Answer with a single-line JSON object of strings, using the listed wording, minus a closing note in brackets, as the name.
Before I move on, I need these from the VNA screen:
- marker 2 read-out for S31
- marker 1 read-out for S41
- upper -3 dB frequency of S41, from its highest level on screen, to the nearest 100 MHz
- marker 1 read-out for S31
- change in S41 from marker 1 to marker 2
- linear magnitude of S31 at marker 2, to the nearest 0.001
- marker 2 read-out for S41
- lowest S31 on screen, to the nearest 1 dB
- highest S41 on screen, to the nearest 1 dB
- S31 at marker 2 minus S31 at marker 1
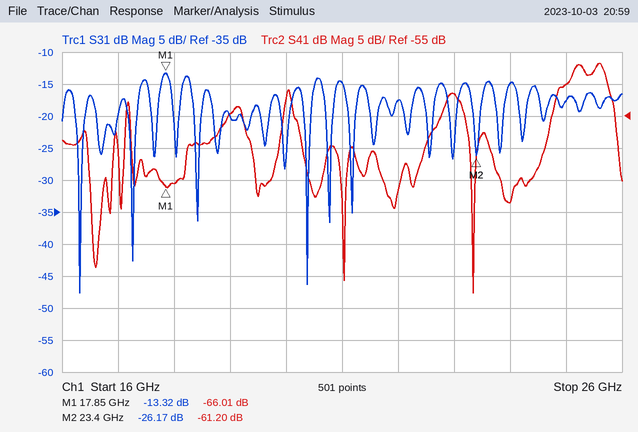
{"marker 2 read-out for S31": "-26.17 dB", "marker 1 read-out for S41": "-66.01 dB", "upper -3 dB frequency of S41, from its highest level on screen, to the nearest 100 MHz": "25.7 GHz", "marker 1 read-out for S31": "-13.32 dB", "change in S41 from marker 1 to marker 2": "4.81 dB", "linear magnitude of S31 at marker 2, to the nearest 0.001": "0.049", "marker 2 read-out for S41": "-61.20 dB", "lowest S31 on screen, to the nearest 1 dB": "-48 dB", "highest S41 on screen, to the nearest 1 dB": "-47 dB", "S31 at marker 2 minus S31 at marker 1": "-12.85 dB"}
